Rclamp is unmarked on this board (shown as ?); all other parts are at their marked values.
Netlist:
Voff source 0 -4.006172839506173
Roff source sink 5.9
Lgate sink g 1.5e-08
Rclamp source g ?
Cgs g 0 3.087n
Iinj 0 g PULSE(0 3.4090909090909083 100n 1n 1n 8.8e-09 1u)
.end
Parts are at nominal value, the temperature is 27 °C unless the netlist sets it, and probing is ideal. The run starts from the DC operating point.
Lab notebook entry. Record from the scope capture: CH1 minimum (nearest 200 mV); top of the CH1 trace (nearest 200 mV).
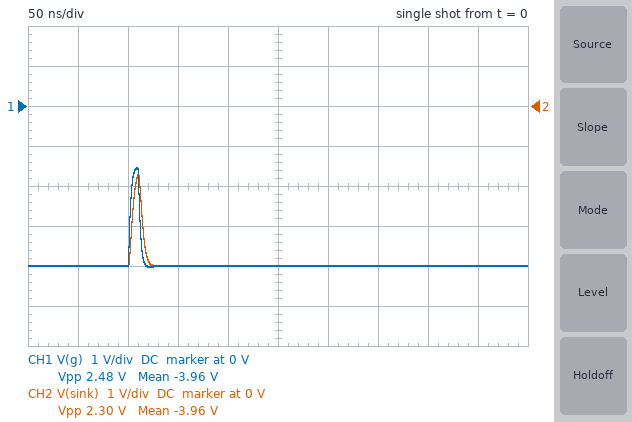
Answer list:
-4.0 V
-1.6 V
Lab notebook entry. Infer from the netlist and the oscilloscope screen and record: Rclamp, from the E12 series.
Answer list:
0.82 Ω
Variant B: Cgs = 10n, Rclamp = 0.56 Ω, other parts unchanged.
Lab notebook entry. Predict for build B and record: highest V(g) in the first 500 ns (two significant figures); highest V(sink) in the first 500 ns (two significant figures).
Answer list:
-2.5 V
-2.7 V
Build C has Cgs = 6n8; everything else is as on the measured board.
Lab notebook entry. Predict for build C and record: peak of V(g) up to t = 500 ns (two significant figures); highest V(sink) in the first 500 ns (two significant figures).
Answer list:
-1.9 V
-2.1 V
